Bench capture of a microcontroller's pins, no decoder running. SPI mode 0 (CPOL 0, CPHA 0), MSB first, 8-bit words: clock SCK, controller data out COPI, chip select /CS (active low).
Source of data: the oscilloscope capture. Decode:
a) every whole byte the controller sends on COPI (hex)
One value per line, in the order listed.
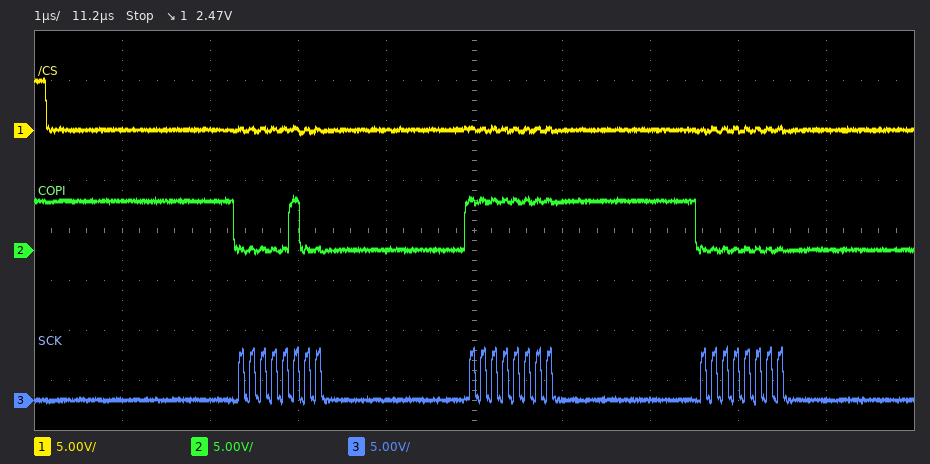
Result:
04 FF 00
